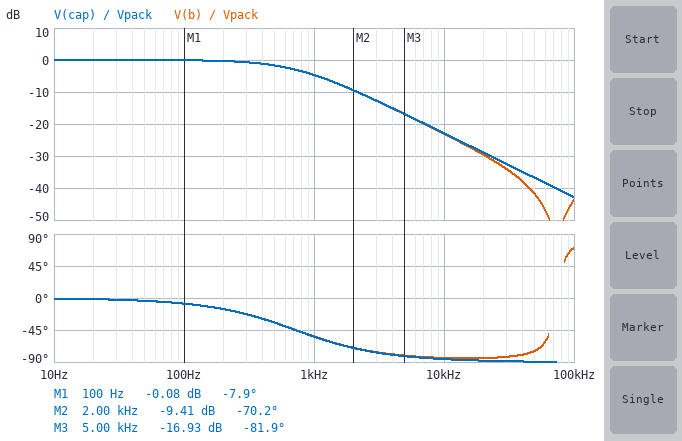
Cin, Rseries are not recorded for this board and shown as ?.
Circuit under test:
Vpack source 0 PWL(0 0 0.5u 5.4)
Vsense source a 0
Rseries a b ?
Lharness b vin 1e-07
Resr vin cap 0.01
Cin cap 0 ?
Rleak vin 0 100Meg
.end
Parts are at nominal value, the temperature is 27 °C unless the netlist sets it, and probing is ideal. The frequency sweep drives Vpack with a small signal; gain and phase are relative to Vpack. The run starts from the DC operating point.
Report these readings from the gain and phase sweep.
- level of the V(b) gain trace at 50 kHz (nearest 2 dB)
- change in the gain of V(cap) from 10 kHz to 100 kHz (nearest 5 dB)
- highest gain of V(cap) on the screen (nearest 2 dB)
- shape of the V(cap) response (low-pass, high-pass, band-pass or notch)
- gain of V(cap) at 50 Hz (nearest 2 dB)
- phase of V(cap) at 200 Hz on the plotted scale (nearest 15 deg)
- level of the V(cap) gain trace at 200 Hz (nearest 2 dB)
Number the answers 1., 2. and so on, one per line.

1. -42 dB
2. -20 dB
3. 0 dB
4. low-pass
5. 0 dB
6. -15 deg
7. 0 dB
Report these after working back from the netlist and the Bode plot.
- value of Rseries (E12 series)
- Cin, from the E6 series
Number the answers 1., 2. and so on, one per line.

1. 4.7 Ω
2. 47 µF
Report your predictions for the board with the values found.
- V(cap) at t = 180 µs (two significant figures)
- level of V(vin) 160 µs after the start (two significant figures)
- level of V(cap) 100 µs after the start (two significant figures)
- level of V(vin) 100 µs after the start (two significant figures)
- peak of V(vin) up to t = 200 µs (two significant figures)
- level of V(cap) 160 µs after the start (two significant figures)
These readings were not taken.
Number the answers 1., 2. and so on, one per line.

1. 3.0 V
2. 2.8 V
3. 2.0 V
4. 2.0 V
5. 3.2 V
6. 2.8 V
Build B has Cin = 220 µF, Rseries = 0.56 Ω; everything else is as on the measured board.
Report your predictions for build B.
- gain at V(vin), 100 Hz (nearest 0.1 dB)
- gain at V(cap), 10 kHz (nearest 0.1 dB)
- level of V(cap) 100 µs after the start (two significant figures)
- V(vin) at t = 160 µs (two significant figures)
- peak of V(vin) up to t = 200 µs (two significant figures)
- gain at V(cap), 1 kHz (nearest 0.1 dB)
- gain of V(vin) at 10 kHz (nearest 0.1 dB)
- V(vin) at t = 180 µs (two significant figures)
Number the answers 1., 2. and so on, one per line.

1. 0 dB
2. -18.0 dB
3. 3.0 V
4. 3.9 V
5. 4.3 V
6. -2.1 dB
7. -17.9 dB
8. 4.1 V
